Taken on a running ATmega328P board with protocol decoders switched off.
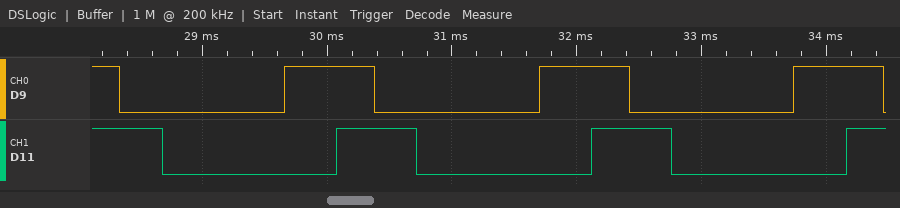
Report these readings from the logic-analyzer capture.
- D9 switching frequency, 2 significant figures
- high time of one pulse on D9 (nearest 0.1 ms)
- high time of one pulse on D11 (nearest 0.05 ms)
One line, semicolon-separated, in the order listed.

490 Hz; 0.7 ms; 0.65 ms
